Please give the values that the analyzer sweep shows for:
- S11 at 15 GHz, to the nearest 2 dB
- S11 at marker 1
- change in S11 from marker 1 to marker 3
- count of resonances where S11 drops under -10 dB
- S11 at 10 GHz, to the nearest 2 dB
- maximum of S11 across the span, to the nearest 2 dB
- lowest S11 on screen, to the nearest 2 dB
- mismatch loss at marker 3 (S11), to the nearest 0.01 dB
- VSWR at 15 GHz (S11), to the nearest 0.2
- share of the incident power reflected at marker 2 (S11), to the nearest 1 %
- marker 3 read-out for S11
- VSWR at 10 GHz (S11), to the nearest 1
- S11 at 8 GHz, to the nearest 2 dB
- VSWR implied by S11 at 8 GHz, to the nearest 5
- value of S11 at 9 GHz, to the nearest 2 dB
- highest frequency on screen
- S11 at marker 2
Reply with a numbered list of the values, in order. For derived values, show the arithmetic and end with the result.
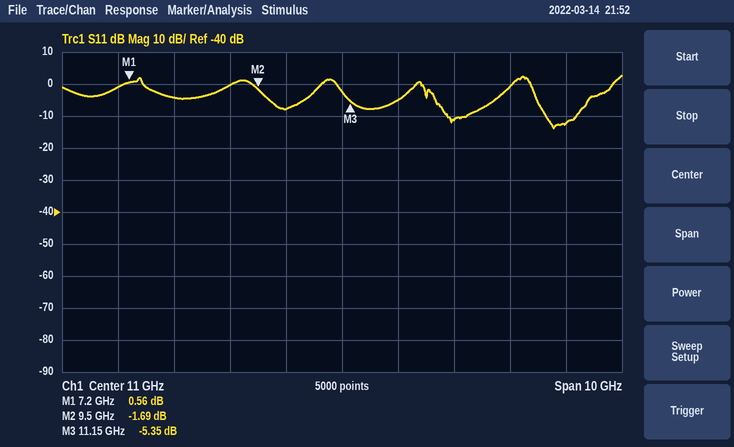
1. -12 dB
2. 0.56 dB
3. -5.35 − (0.56) = -5.91 dB
4. 2
5. -8 dB
6. 2 dB
7. -14 dB
8. −10 log10(1 − 10^(-5.35/10)) ≈ 1.50 dB
9. |Γ| = 10^(-12/20) = 0.2512; VSWR = (1 + 0.2512)/(1 − 0.2512) ≈ 1.67, so 1.6 to the nearest 0.2
10. 10^(-1.69/10) ≈ 68 %
11. -5.35 dB
12. |Γ| = 10^(-8/20) = 0.3981; VSWR = (1 + 0.3981)/(1 − 0.3981) ≈ 2
13. -4 dB
14. |Γ| = 10^(-4/20) = 0.6310; VSWR = (1 + 0.6310)/(1 − 0.6310) ≈ 4.42, so 5 to the nearest 5
15. 0 dB
16. 16 GHz
17. -1.69 dB
